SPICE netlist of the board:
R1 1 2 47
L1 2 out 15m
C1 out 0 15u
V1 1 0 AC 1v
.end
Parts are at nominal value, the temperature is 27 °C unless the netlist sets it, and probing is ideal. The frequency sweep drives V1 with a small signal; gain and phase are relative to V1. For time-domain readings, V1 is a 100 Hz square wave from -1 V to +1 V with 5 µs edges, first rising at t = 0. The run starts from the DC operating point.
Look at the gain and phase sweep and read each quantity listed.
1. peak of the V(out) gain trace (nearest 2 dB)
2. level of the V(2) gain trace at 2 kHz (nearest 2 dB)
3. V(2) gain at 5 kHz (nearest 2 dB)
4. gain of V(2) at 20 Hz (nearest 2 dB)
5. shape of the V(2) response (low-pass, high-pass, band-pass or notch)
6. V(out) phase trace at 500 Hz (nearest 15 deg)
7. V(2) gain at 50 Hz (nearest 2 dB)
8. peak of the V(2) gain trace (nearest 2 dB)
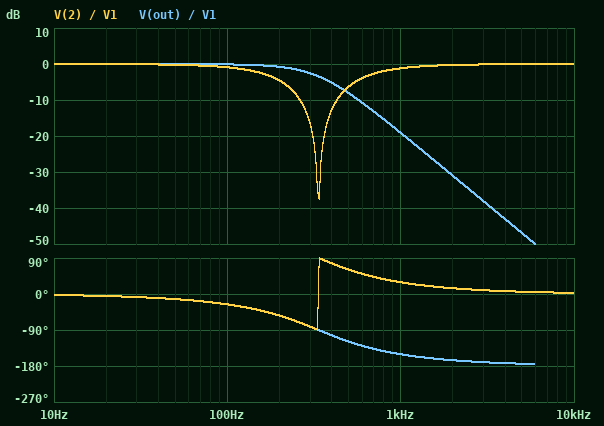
0 dB
0 dB
0 dB
0 dB
notch
-120 deg
0 dB
0 dB
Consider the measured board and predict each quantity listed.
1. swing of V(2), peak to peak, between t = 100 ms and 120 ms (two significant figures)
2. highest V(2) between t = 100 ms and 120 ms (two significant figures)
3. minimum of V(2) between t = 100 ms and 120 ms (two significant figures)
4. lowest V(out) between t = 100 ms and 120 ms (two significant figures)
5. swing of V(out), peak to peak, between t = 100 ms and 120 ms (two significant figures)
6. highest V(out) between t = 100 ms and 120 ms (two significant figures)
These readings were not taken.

2.1 V
1.0 V
-1.0 V
-1.1 V
2.1 V
1.1 V
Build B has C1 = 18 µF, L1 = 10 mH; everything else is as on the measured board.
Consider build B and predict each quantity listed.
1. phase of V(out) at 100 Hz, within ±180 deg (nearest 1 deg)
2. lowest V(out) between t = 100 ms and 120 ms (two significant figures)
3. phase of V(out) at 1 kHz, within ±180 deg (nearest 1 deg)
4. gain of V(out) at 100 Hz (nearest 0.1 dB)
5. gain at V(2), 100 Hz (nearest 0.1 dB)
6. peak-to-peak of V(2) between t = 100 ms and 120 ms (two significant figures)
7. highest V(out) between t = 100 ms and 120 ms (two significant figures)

-30 deg
-1.0 V
-139 deg
-0.6 dB
-1.2 dB
2.0 V
1.0 V
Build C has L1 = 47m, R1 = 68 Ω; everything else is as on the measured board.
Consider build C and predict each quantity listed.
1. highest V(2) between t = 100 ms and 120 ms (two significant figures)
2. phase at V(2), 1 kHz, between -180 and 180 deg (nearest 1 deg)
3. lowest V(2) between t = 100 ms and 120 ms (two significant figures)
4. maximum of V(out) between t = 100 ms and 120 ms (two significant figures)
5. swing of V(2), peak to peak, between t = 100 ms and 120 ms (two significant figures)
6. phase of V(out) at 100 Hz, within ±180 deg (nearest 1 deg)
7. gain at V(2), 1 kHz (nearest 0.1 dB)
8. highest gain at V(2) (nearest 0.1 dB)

1.1 V
13 deg
-1.1 V
1.2 V
2.2 V
-42 deg
-0.2 dB
0 dB
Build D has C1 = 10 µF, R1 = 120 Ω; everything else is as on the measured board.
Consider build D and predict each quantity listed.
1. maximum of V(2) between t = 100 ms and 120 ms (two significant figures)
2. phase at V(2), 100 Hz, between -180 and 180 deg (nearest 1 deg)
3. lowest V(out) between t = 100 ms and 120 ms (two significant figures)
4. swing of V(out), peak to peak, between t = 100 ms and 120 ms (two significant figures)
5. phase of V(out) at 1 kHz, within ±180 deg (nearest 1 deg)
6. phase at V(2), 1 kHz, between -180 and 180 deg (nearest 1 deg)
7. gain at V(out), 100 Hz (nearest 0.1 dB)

980 mV
-39 deg
-980 mV
2.0 V
-123 deg
57 deg
-1.6 dB
